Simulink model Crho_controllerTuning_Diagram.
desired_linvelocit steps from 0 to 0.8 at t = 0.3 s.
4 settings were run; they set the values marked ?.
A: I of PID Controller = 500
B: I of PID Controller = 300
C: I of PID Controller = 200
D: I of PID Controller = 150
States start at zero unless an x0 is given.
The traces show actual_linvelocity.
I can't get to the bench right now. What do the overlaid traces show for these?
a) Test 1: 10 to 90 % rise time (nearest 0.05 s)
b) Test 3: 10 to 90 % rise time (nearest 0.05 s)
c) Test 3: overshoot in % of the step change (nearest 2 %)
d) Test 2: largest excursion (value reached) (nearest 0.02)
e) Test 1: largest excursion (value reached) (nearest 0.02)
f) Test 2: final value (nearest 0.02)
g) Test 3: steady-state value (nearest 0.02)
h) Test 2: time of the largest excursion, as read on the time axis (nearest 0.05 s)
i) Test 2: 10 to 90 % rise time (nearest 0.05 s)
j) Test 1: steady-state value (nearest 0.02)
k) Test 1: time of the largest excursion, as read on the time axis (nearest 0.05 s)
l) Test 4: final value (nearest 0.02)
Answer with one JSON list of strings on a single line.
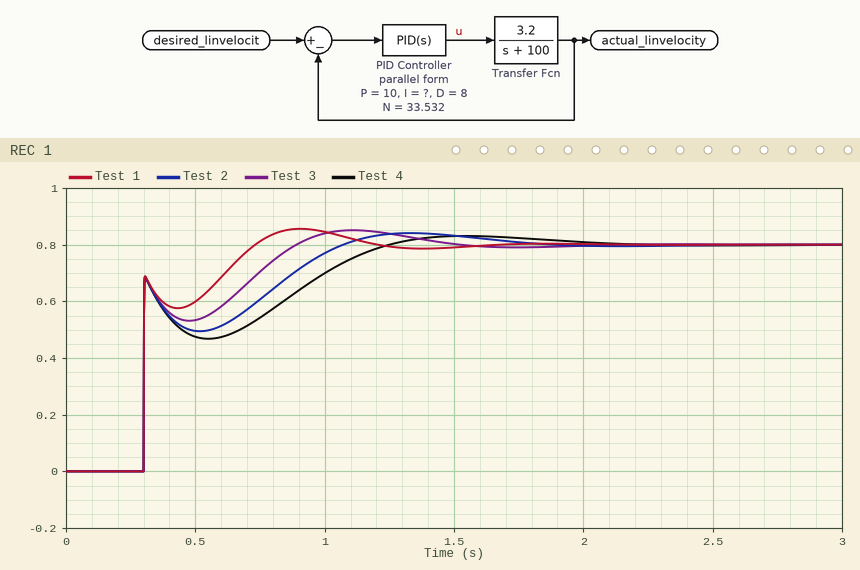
["0.35 s", "0.45 s", "6 %", "0.84", "0.86", "0.80", "0.80", "1.35 s", "0.60 s", "0.80", "0.90 s", "0.80"]
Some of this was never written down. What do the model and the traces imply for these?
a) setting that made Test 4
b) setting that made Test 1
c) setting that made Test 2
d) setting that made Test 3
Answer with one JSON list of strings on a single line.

["D", "A", "C", "B"]
